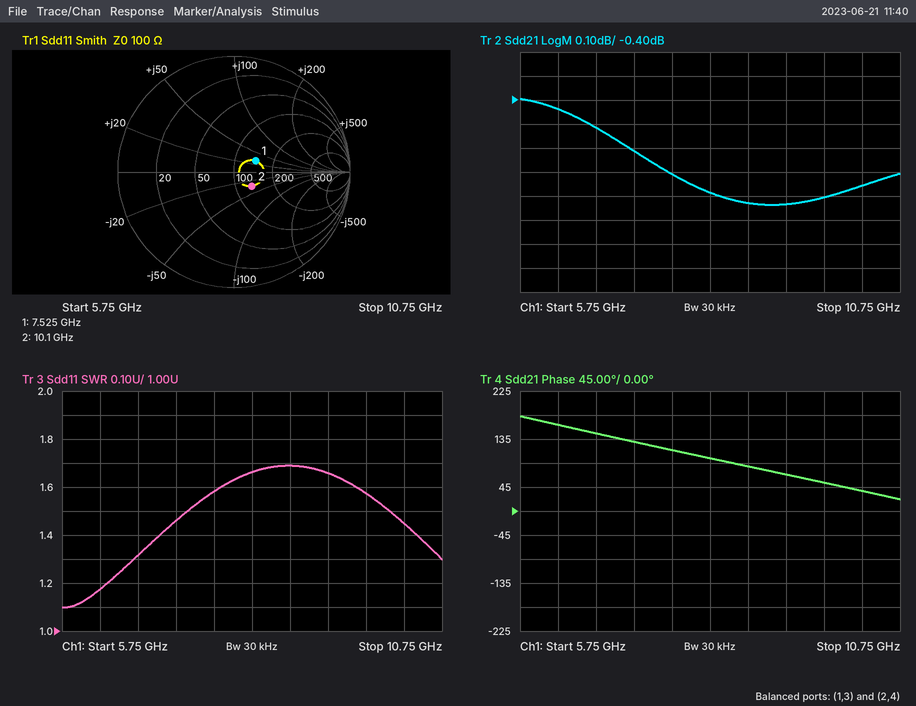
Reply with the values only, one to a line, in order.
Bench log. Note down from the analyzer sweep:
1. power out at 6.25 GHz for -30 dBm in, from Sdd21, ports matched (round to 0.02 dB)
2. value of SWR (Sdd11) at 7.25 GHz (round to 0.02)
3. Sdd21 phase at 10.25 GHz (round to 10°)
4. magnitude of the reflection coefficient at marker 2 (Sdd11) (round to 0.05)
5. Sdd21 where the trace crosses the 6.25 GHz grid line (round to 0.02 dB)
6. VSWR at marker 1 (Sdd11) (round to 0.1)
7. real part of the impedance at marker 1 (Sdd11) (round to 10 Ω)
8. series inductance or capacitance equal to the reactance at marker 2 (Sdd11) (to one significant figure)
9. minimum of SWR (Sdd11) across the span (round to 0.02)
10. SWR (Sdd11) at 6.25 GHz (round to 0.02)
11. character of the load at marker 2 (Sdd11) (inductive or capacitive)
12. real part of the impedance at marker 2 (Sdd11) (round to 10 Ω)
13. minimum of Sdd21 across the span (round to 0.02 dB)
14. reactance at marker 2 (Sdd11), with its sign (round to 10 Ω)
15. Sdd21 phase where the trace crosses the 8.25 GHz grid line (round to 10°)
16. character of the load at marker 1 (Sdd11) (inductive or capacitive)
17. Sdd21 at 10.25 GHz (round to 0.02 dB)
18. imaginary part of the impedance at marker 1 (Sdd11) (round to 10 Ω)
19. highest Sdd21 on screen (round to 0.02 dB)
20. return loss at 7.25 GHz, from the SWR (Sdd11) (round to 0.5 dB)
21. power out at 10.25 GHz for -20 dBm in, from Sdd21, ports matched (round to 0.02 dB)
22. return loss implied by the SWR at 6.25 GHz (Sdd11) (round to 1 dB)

-30.44 dBm
1.46
40°
0.20
-0.44 dB
1.5
140 Ω
500 fF
1.10
1.18
capacitive
130 Ω
-0.84 dB
-30 Ω
100°
inductive
-0.76 dB
+30 Ω
-0.40 dB
14.5 dB
-20.76 dBm
22 dB
